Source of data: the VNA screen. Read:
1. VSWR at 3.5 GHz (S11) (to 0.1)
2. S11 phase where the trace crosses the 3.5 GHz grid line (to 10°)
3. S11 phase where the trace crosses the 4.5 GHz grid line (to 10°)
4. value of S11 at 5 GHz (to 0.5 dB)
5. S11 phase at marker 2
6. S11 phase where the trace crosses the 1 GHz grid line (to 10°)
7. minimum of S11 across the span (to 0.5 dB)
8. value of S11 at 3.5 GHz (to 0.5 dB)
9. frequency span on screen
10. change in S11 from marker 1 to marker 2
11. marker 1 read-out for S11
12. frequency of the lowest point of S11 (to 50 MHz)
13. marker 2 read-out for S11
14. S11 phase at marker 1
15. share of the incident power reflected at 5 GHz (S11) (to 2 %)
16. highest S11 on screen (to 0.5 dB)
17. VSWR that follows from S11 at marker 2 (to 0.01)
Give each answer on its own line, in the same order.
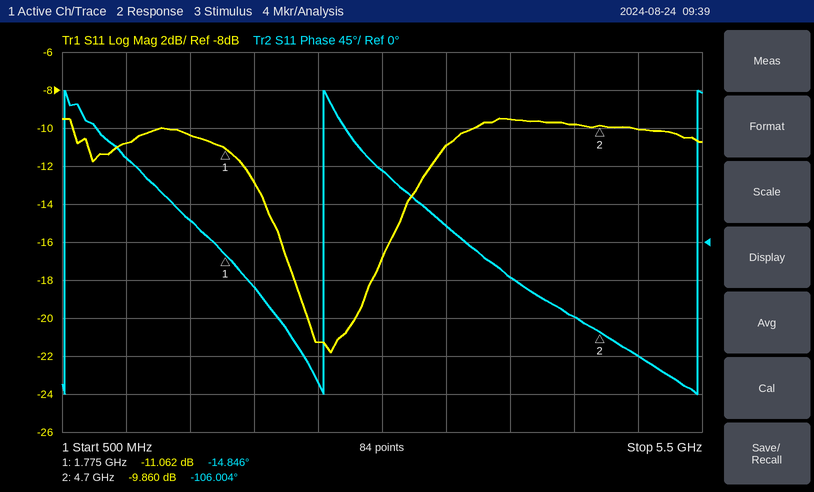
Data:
1.8
20°
-90°
-10.0 dB
-106.004°
100°
-22.0 dB
-11.0 dB
5 GHz
1.202 dB
-11.062 dB
2.60 GHz
-9.860 dB
-14.846°
10 %
-9.5 dB
1.95
